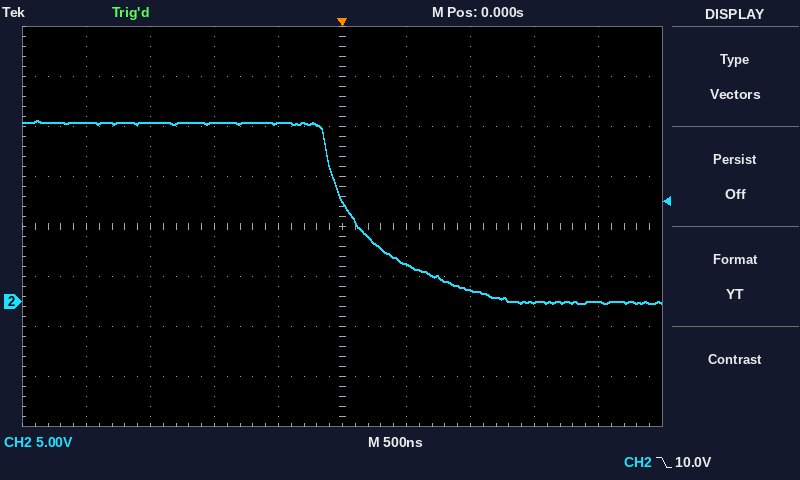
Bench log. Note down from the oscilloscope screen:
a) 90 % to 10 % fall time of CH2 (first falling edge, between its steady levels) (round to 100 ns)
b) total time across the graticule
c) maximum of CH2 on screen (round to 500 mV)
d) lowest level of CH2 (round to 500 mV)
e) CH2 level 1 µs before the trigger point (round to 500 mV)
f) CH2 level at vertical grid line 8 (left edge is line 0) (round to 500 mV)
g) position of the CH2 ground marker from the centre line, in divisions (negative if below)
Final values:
1.0 µs
5 µs
18.0 V
0.0 V
18.0 V
0.0 V
-1.5 div
